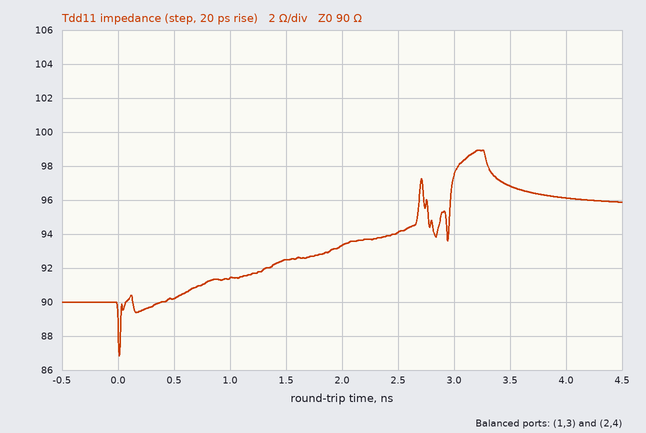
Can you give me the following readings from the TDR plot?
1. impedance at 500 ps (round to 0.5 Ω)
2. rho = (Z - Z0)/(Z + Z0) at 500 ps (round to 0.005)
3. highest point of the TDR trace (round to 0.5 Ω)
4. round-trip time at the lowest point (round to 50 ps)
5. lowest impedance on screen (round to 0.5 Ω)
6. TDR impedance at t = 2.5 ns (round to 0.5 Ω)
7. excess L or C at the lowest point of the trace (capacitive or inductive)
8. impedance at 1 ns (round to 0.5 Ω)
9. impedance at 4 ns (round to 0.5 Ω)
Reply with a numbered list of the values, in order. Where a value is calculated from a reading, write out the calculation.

1. 90.0 Ω
2. (90 − 90)/(90 + 90) ≈ 0.000
3. 99.0 Ω
4. 0 ps
5. 87.0 Ω
6. 94.0 Ω
7. capacitive
8. 91.5 Ω
9. 96.0 Ω
